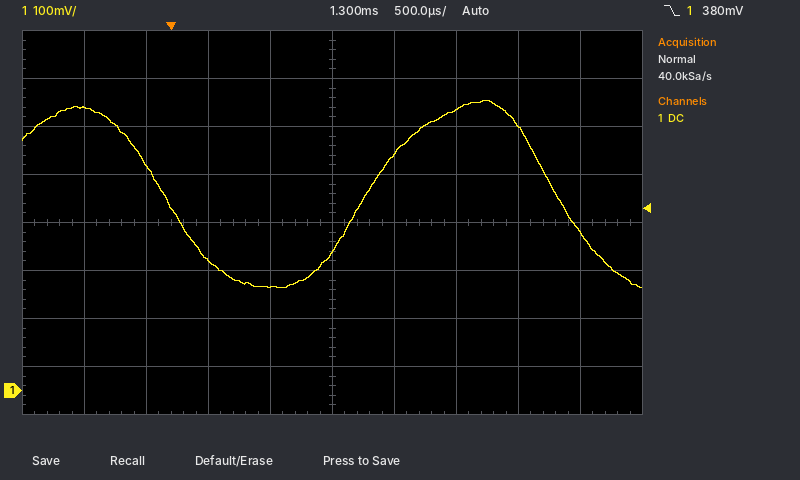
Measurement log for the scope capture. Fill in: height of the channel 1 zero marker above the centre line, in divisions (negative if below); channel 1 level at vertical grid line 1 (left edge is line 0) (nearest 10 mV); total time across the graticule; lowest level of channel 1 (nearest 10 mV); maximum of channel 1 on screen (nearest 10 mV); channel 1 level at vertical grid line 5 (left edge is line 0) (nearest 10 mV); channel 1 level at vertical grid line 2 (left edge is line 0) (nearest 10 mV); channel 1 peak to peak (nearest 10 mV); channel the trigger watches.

-3.5 div
590 mV
5 ms
210 mV
600 mV
290 mV
470 mV
390 mV
channel 1
